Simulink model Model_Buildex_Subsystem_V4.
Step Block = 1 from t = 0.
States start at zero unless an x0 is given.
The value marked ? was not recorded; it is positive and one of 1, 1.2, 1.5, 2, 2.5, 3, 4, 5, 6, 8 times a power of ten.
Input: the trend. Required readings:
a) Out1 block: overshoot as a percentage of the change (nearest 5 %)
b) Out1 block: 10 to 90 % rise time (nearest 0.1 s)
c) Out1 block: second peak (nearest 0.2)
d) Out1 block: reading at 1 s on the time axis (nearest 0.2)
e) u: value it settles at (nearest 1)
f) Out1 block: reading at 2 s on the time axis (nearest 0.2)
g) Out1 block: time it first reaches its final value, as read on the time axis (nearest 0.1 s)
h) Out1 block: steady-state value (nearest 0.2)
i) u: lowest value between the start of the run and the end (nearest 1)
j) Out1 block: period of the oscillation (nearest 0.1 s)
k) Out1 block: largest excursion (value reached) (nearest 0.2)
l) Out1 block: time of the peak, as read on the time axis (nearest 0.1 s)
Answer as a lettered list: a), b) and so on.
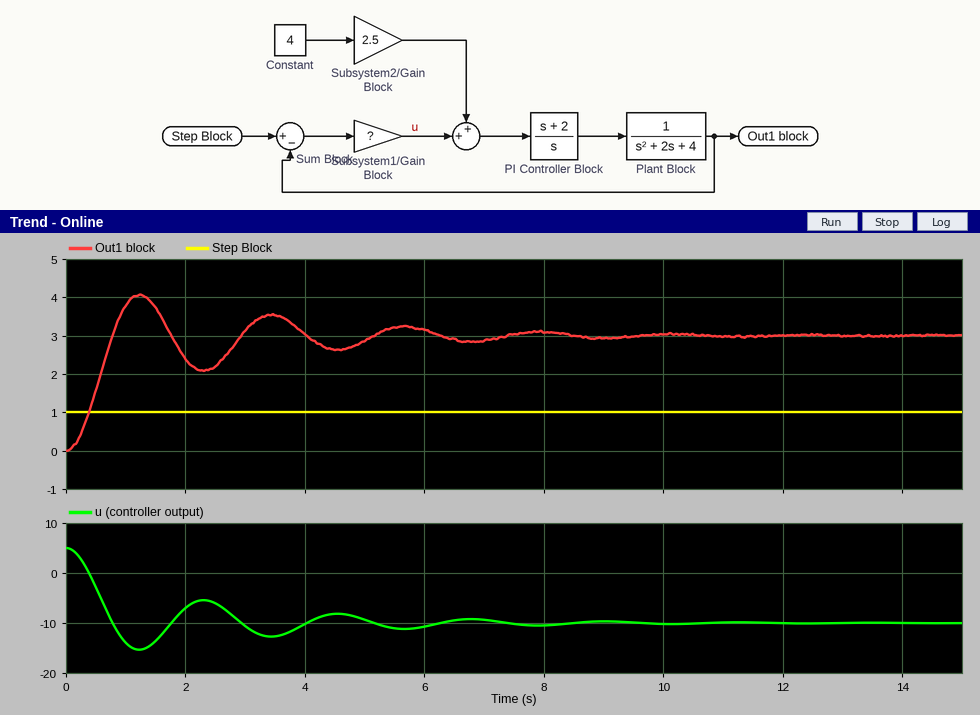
a) 35 %
b) 0.5 s
c) 3.6
d) 3.8
e) -10
f) 2.4
g) 0.8 s
h) 3.0
i) -15
j) 2.2 s
k) 4.0
l) 1.2 s
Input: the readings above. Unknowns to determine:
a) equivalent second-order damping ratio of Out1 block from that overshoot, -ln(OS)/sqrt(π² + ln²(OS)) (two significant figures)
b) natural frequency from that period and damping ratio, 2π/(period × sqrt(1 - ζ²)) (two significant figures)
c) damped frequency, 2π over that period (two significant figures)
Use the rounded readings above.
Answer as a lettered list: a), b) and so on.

a) 0.32
b) 3.0 rad/s
c) 2.9 rad/s
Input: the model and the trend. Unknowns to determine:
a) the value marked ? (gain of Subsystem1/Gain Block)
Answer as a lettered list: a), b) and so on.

a) 5
